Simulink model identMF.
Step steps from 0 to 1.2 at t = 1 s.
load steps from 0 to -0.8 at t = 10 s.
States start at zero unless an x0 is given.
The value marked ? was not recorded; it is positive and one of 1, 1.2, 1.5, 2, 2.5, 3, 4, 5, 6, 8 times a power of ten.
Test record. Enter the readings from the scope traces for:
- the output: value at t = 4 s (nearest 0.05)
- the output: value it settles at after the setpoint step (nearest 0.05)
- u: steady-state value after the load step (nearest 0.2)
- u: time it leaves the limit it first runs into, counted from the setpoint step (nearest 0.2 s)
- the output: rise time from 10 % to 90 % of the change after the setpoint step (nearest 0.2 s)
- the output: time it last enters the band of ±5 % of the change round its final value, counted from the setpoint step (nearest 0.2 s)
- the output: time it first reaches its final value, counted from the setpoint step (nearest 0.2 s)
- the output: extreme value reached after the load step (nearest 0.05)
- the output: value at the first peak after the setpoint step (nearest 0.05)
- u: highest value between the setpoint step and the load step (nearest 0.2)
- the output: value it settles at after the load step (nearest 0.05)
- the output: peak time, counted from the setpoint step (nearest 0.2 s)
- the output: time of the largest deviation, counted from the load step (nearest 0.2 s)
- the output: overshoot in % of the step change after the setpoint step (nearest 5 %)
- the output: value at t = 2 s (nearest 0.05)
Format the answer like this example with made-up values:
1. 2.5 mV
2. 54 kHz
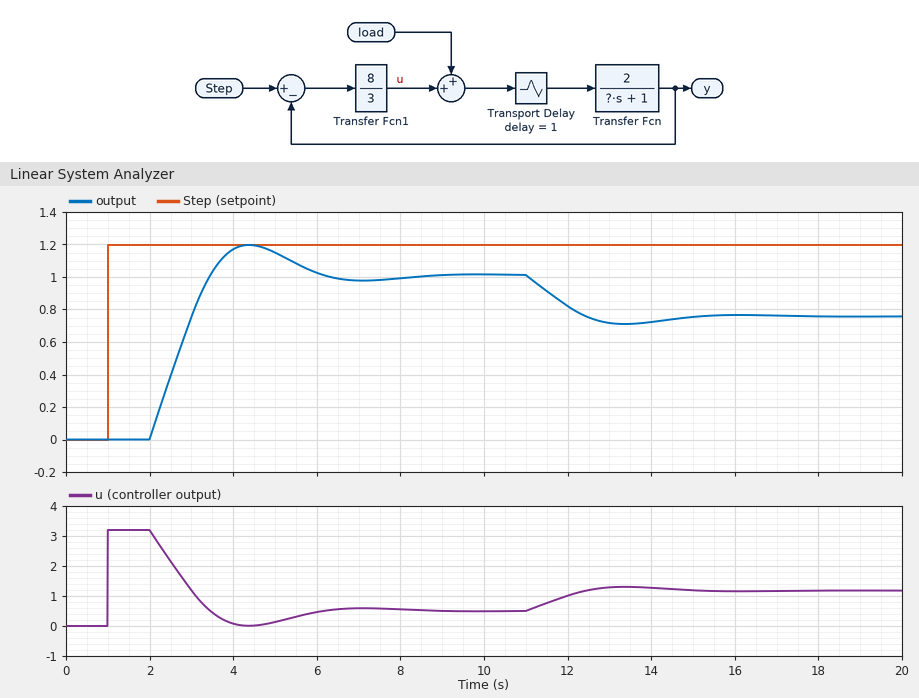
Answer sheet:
1. 1.15
2. 1.00
3. 1.2
4. 1.0 s
5. 1.2 s
6. 4.6 s
7. 2.4 s
8. 0.70
9. 1.20
10. 3.2
11. 0.75
12. 3.4 s
13. 3.4 s
14. 20 %
15. 0.00
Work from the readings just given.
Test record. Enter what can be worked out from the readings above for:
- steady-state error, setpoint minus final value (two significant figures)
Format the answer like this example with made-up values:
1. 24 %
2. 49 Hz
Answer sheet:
1. 0.20
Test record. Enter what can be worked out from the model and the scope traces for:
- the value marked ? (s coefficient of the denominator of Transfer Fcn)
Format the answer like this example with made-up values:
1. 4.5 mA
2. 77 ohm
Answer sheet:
1. 8
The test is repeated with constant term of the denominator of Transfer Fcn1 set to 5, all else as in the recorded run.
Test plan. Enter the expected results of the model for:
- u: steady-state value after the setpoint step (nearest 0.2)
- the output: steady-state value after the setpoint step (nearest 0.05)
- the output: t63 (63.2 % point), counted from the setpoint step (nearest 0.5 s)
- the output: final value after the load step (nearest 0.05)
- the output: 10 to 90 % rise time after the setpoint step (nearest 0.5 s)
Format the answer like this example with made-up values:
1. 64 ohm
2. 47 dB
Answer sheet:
1. 0.4
2. 0.90
3. 2.5 s
4. 0.55
5. 2.0 s
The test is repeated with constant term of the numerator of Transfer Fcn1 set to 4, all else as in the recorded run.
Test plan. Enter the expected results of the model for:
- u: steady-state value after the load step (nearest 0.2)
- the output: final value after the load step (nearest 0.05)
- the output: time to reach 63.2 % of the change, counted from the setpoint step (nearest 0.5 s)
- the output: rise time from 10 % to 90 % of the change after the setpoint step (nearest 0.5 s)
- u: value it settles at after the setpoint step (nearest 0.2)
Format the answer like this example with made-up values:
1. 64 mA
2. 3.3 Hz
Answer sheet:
1. 1.0
2. 0.45
3. 2.5 s
4. 3.0 s
5. 0.4
